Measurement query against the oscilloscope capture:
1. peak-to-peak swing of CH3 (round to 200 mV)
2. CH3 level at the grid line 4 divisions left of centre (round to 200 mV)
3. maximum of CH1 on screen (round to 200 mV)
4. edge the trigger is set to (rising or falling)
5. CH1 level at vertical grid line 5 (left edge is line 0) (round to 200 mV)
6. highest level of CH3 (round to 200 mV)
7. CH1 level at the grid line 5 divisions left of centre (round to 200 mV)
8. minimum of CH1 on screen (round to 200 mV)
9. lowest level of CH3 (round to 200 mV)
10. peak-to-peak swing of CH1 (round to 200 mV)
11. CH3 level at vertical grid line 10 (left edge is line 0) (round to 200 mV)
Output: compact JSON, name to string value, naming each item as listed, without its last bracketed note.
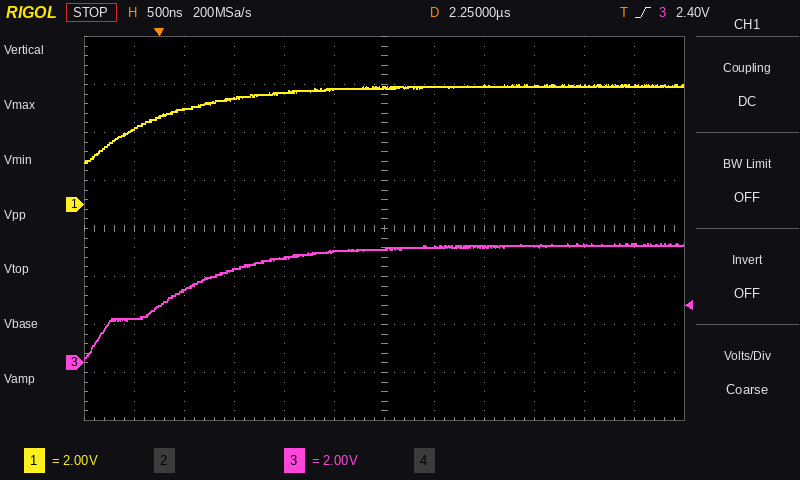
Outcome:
{"peak-to-peak swing of CH3": "4.8 V", "CH3 level at the grid line 4 divisions left of centre": "3.0 V", "maximum of CH1 on screen": "5.0 V", "edge the trigger is set to": "rising", "CH1 level at vertical grid line 5 (left edge is line 0)": "4.8 V", "highest level of CH3": "5.0 V", "CH1 level at the grid line 5 divisions left of centre": "3.2 V", "minimum of CH1 on screen": "1.8 V", "lowest level of CH3": "200 mV", "peak-to-peak swing of CH1": "3.2 V", "CH3 level at vertical grid line 10 (left edge is line 0)": "5.0 V"}
